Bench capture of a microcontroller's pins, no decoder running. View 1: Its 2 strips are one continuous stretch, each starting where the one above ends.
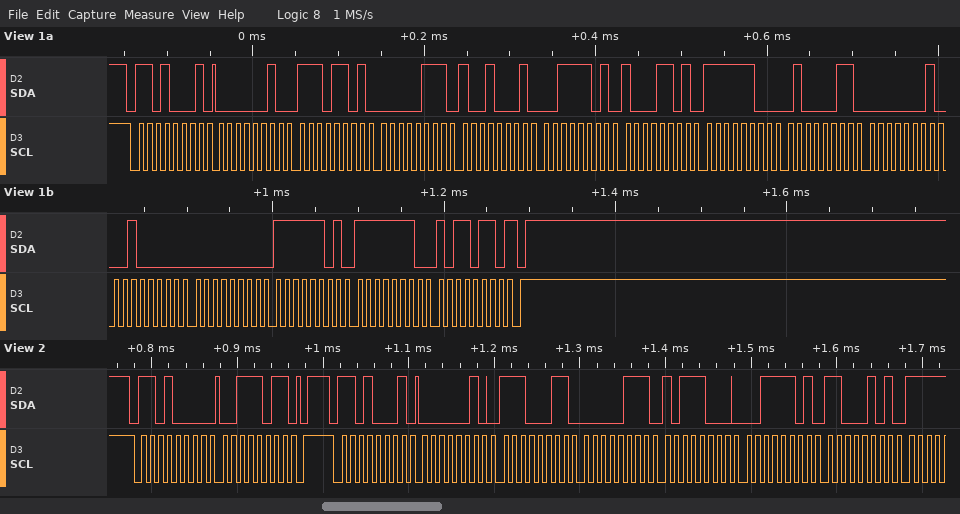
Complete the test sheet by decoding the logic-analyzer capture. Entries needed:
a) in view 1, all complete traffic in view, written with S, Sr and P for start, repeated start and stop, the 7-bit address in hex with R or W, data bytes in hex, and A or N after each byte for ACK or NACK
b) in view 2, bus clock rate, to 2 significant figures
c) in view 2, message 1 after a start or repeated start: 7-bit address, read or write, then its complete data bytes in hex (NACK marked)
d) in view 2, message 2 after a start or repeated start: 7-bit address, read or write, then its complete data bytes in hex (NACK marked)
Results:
S 68R A 02 A ED A 07 A 91 A 3D A 8D A FC A 43 A 01 A 20 A 00 A FD A FE A B6 N P
100 kHz
0x68 write: 3B
0x68 read: 02 E3 07 B8 3D C5
